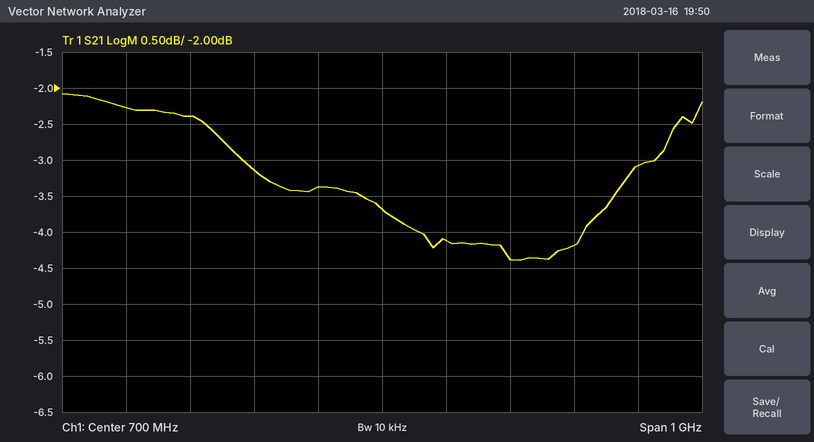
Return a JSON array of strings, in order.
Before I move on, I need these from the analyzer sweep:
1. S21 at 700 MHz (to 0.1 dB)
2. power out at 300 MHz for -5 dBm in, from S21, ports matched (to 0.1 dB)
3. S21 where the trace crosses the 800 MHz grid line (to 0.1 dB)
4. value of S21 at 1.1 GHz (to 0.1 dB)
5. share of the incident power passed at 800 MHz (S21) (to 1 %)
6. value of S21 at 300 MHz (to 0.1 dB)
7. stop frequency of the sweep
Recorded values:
["-3.7 dB", "-7.3 dBm", "-4.1 dB", "-3.1 dB", "39 %", "-2.3 dB", "1.2 GHz"]
